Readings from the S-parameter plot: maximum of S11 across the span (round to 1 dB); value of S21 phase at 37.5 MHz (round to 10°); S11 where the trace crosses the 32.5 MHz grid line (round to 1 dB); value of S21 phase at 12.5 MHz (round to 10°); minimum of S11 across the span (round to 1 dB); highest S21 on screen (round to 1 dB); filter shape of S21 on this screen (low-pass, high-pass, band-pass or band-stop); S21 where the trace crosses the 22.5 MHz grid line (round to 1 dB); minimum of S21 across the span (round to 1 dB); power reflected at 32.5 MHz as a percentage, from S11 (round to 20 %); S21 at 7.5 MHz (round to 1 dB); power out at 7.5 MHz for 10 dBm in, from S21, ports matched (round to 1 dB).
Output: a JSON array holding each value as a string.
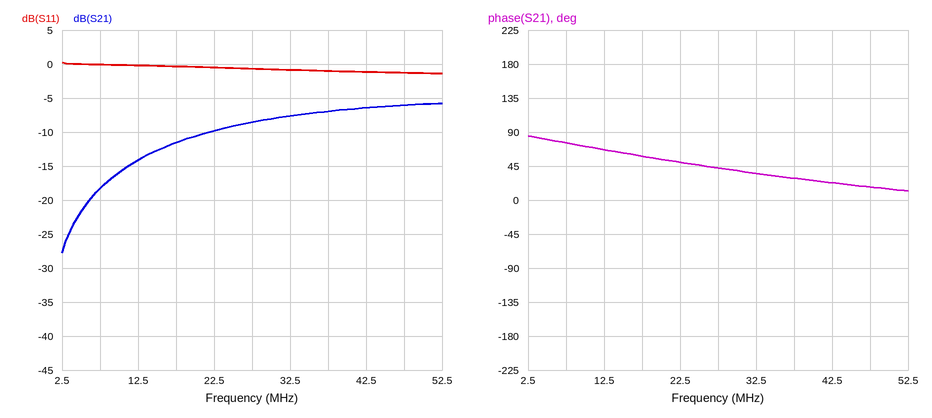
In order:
["0 dB", "30°", "-1 dB", "70°", "-1 dB", "-6 dB", "high-pass", "-10 dB", "-28 dB", "80 %", "-18 dB", "-8 dBm"]
